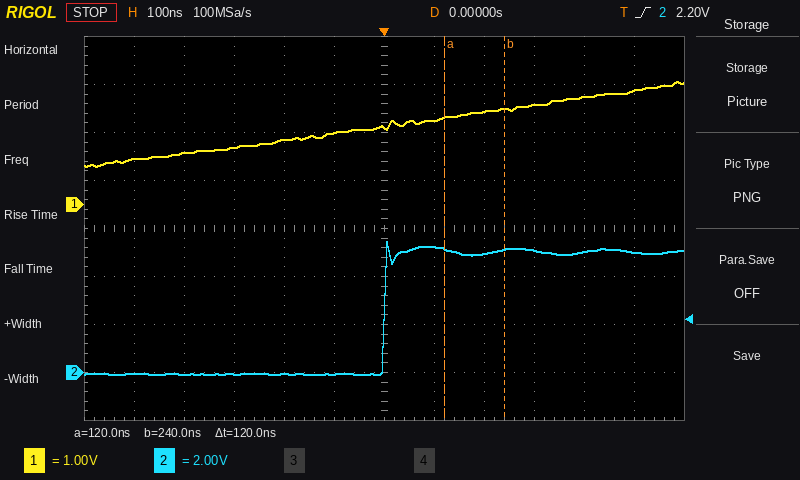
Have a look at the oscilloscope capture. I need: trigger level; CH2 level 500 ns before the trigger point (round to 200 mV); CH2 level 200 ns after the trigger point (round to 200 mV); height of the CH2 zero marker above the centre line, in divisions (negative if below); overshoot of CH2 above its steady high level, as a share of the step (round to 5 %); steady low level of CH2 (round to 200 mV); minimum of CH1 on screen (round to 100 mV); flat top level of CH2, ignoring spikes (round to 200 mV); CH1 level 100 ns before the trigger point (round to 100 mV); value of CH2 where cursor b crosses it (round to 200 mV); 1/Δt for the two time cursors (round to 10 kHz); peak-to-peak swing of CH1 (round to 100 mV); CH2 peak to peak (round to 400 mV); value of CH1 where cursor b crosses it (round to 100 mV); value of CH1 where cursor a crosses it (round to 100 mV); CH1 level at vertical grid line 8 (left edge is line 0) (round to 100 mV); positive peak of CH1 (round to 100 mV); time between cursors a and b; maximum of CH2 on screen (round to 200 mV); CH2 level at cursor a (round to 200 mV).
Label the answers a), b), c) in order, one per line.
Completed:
a) 2.20 V
b) 0.0 V
c) 5.0 V
d) -3.0 div
e) 10 %
f) 0.0 V
g) 800 mV
h) 5.0 V
i) 1.5 V
j) 5.2 V
k) 8.33 MHz
l) 1.8 V
m) 5.6 V
n) 2.0 V
o) 1.8 V
p) 1.9 V
q) 2.6 V
r) 120 ns
s) 5.4 V
t) 5.2 V
